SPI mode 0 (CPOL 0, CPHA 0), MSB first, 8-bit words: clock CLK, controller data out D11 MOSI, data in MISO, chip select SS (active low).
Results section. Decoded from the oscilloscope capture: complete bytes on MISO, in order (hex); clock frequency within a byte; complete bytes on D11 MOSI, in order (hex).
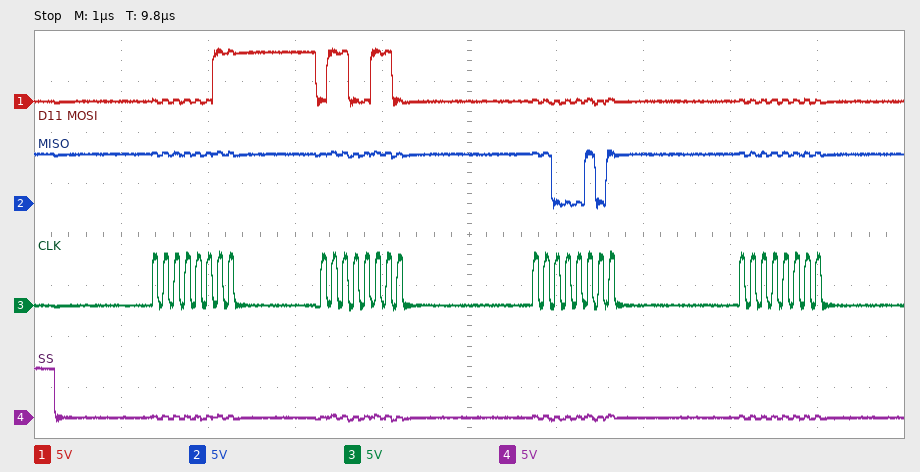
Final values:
FF FF C5 FF
8 MHz
03 66 00 00
